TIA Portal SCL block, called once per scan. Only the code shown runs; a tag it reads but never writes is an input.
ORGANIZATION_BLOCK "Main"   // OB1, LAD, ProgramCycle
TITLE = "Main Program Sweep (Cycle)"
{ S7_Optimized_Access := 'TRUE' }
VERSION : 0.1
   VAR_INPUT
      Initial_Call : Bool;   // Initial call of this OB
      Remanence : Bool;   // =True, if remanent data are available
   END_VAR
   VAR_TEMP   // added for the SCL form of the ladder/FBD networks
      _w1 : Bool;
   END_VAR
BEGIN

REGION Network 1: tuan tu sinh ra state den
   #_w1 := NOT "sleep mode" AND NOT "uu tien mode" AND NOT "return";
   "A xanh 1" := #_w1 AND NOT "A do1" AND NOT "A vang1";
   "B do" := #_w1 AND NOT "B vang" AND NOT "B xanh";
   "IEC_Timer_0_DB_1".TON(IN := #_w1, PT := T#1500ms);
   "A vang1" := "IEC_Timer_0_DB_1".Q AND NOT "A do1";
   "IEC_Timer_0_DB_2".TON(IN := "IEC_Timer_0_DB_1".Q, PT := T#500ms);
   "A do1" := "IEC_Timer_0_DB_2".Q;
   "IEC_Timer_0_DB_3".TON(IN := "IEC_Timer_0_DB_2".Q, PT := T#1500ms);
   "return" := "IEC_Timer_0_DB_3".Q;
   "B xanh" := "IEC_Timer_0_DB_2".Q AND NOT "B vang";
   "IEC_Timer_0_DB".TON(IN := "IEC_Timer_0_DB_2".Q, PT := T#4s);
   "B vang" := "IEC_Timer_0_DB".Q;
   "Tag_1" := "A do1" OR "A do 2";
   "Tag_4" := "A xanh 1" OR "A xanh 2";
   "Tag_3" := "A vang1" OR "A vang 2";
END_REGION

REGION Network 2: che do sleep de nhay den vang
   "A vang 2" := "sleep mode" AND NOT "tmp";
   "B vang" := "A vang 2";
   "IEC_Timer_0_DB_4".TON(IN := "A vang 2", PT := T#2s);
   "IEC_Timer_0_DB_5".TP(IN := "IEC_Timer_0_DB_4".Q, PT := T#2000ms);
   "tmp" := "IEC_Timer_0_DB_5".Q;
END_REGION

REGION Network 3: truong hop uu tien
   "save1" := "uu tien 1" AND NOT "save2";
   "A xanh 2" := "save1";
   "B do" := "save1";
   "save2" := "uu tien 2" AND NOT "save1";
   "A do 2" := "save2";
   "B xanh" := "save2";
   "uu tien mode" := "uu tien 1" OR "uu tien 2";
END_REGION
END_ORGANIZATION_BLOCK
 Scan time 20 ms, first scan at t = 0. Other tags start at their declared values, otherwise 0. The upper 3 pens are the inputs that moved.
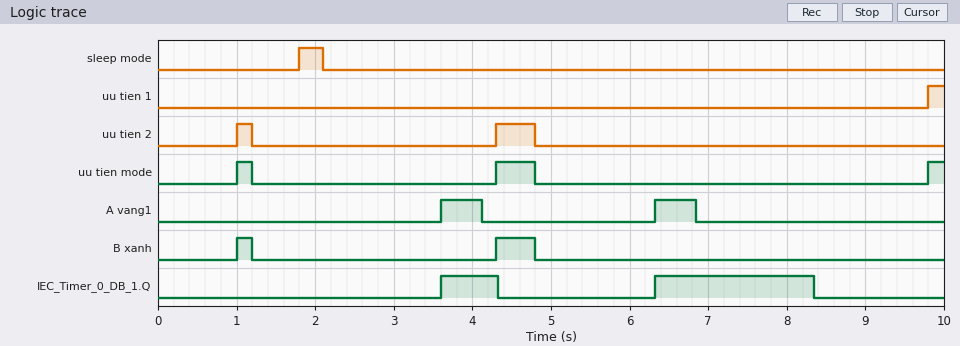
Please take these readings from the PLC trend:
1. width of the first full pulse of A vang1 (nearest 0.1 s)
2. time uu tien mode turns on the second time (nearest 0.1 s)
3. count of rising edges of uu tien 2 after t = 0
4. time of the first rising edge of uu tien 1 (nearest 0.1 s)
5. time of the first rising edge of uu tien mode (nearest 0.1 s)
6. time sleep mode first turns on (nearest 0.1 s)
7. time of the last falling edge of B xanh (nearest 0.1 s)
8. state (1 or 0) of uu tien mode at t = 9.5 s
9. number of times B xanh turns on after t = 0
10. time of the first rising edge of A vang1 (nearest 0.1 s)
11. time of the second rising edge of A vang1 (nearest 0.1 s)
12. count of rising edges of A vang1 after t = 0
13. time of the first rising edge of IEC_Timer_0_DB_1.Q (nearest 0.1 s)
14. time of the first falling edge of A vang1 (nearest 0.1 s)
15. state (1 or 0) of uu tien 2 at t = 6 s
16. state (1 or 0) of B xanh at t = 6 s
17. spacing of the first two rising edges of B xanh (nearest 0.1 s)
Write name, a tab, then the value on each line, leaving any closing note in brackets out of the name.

width of the first full pulse of A vang1	0.5 s
time uu tien mode turns on the second time	4.3 s
count of rising edges of uu tien 2 after t = 0	2
time of the first rising edge of uu tien 1	9.8 s
time of the first rising edge of uu tien mode	1.0 s
time sleep mode first turns on	1.8 s
time of the last falling edge of B xanh	4.8 s
state (1 or 0) of uu tien mode at t = 9.5 s	0
number of times B xanh turns on after t = 0	2
time of the first rising edge of A vang1	3.6 s
time of the second rising edge of A vang1	6.3 s
count of rising edges of A vang1 after t = 0	2
time of the first rising edge of IEC_Timer_0_DB_1.Q	3.6 s
time of the first falling edge of A vang1	4.1 s
state (1 or 0) of uu tien 2 at t = 6 s	0
state (1 or 0) of B xanh at t = 6 s	0
spacing of the first two rising edges of B xanh	3.3 s
